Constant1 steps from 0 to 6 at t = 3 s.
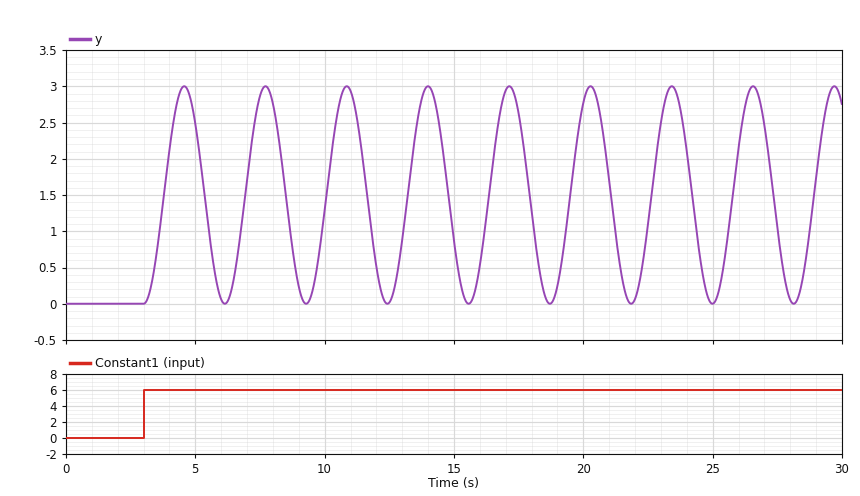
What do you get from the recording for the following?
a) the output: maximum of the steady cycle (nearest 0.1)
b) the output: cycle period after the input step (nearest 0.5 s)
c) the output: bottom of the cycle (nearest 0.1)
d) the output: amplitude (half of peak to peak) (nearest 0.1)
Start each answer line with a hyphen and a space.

- 3.0
- 3.0 s
- 0.0
- 1.5
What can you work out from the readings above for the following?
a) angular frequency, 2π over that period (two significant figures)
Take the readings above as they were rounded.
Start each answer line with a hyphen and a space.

- 2.1 rad/s
